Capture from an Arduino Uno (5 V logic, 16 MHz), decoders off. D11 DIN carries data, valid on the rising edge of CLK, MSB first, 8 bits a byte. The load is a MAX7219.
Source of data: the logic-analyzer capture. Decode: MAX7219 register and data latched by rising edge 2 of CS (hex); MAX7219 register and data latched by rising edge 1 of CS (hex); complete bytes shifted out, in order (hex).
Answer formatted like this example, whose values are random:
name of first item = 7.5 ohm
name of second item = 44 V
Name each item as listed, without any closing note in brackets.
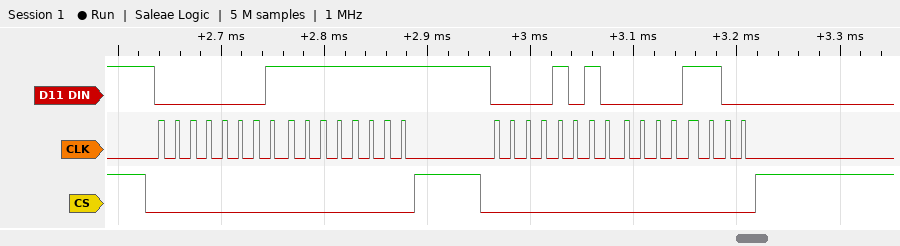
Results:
MAX7219 register and data latched by rising edge 2 of CS = register 0xA, data 0x0C
MAX7219 register and data latched by rising edge 1 of CS = register 0x1, data 0xFF
complete bytes shifted out, in order = 01 FF 0A 0C
